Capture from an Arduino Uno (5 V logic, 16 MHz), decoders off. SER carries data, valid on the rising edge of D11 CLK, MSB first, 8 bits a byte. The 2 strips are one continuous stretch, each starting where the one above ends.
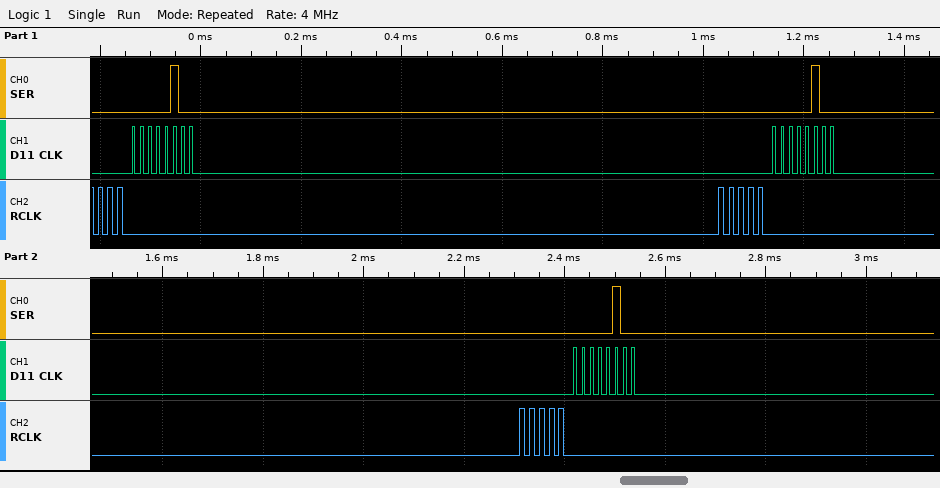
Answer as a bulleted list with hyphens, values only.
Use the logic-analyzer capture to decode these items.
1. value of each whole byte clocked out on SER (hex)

- 04 04 04
